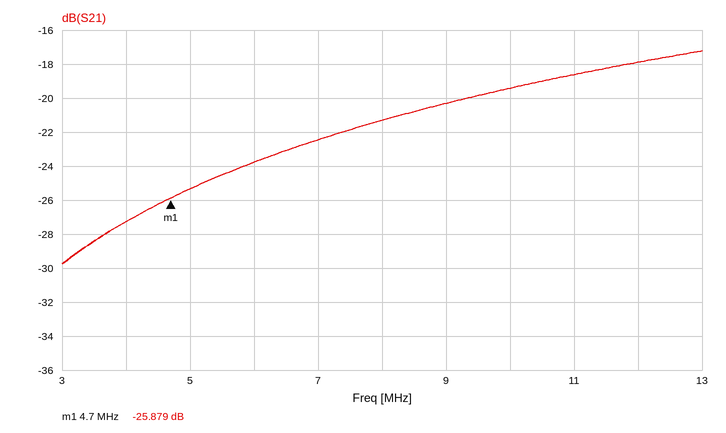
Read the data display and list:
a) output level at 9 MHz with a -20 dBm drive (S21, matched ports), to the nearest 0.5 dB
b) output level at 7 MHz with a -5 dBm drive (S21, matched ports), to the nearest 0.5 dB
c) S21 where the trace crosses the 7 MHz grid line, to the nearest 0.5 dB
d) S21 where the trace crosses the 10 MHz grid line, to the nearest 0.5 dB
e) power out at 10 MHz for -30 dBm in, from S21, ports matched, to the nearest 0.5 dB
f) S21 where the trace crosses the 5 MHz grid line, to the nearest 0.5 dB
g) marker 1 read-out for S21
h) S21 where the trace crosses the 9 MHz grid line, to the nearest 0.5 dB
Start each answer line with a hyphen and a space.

- -40.5 dBm
- -27.5 dBm
- -22.5 dB
- -19.5 dB
- -49.5 dBm
- -25.5 dB
- -25.879 dB
- -20.5 dB
